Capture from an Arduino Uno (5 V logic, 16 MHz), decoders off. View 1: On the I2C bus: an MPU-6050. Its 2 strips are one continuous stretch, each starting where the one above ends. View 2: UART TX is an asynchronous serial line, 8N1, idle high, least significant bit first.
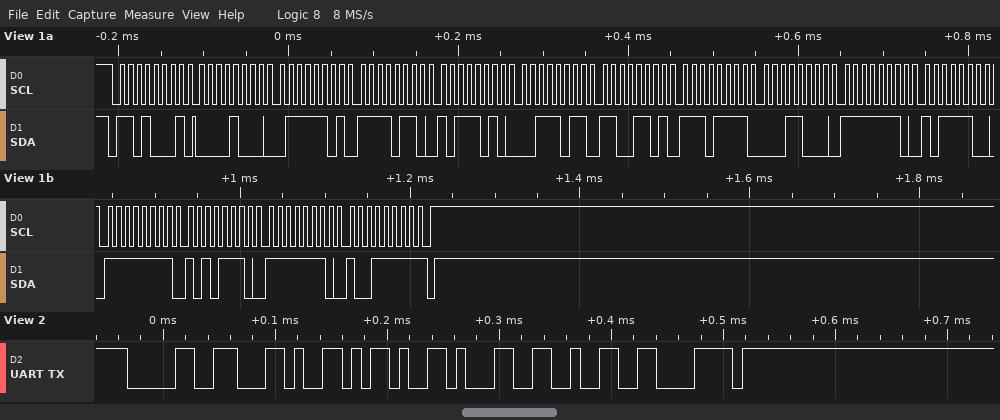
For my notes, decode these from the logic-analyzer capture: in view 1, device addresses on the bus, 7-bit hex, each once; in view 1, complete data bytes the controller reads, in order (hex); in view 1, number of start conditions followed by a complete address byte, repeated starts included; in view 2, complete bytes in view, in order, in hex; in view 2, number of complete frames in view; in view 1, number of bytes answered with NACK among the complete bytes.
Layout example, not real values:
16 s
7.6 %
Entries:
0x68
08 7D F6 BA 3B CD EF 18 FE BC FF AE FE 9F
1
30 2C 2D 31 32 78
6
1
